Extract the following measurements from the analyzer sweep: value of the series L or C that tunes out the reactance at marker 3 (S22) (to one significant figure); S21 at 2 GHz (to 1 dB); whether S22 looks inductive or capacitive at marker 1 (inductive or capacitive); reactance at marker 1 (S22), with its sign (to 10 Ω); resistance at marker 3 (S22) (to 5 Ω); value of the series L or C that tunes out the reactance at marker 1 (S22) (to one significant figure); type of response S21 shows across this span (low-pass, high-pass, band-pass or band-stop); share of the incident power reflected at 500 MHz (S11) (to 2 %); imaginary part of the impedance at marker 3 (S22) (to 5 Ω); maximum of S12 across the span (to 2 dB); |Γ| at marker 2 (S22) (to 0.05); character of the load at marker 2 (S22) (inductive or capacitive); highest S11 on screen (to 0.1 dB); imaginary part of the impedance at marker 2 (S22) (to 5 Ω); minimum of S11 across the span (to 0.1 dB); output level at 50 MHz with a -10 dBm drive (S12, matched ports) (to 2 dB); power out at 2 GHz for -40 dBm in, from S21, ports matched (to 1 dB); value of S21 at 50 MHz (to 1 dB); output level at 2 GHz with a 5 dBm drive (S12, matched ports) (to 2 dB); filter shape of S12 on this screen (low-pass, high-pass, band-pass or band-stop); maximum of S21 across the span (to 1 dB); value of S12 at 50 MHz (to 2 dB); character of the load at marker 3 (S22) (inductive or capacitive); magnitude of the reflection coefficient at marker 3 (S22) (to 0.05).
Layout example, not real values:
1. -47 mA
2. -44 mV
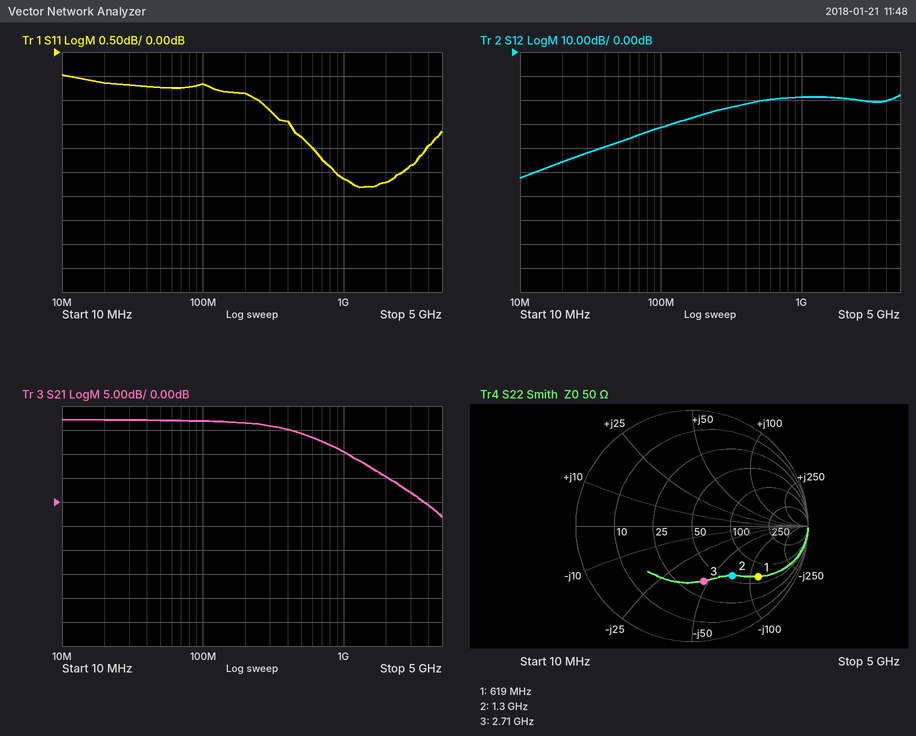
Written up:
1. 3 nH
2. 5 dB
3. capacitive
4. -120 Ω
5. 35 Ω
6. 30 nH
7. low-pass
8. 66 %
9. -45 Ω
10. -18 dB
11. 0.55
12. capacitive
13. -0.5 dB
14. -70 Ω
15. -2.8 dB
16. -48 dBm
17. -35 dBm
18. 17 dB
19. -14 dBm
20. high-pass
21. 17 dB
22. -38 dB
23. capacitive
24. 0.50
